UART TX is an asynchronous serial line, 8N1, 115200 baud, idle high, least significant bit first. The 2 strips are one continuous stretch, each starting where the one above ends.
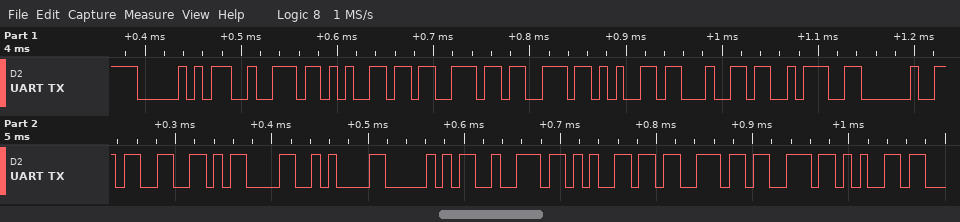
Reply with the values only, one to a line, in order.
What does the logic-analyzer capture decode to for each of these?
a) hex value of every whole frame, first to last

0x50 0x72 0x65 0x73 0x73 0x65 0x64 0x3A 0x20 0x33 0x0D 0x0A 0x50 0x72 0x65 0x73 0x73 0x65
